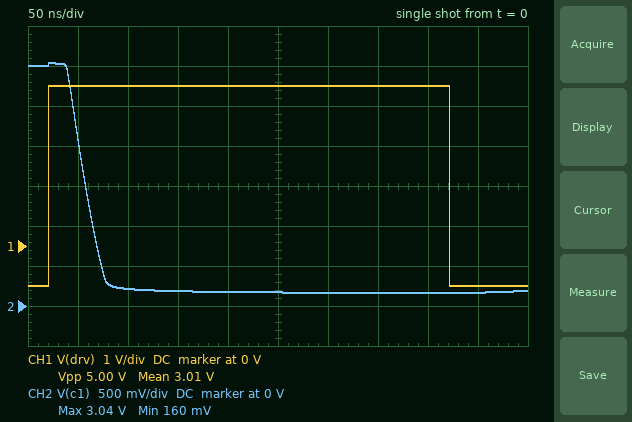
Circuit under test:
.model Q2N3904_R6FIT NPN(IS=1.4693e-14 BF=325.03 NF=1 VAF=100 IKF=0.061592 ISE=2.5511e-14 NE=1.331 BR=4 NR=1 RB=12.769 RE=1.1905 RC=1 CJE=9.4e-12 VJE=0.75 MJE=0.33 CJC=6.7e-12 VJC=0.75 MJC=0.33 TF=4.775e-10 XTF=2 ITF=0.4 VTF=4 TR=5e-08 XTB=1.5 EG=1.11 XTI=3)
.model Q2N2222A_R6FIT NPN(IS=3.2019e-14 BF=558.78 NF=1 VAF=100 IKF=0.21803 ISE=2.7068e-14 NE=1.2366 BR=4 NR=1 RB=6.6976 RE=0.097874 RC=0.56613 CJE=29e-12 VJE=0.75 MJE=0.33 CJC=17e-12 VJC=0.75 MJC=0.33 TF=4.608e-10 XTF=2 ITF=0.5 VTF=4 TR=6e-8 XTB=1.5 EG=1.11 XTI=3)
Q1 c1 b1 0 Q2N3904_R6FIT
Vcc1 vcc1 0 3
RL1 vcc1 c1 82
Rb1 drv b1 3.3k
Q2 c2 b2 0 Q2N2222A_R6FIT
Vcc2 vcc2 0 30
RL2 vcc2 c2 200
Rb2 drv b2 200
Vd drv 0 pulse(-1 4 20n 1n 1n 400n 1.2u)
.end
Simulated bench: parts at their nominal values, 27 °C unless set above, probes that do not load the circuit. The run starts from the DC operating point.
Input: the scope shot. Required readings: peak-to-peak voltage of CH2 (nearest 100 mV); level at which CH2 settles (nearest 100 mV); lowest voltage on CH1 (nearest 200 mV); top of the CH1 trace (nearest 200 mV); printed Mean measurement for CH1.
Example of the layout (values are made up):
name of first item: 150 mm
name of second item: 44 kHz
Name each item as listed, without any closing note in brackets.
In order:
peak-to-peak voltage of CH2: 2.9 V
level at which CH2 settles: 200 mV
lowest voltage on CH1: -1.0 V
top of the CH1 trace: 4.0 V
printed Mean measurement for CH1: 3.01 V
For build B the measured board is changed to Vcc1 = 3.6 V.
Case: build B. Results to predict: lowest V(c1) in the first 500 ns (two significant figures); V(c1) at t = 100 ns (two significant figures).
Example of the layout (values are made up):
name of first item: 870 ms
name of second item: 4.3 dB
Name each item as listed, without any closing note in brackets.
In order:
lowest V(c1) in the first 500 ns: 180 mV
V(c1) at t = 100 ns: 250 mV
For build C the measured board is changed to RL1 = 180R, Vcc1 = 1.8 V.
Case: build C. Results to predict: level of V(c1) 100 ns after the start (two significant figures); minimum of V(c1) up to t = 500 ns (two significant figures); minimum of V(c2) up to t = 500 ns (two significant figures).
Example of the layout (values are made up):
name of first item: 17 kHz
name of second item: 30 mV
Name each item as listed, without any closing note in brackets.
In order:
level of V(c1) 100 ns after the start: 97 mV
minimum of V(c1) up to t = 500 ns: 60 mV
minimum of V(c2) up to t = 500 ns: 150 mV
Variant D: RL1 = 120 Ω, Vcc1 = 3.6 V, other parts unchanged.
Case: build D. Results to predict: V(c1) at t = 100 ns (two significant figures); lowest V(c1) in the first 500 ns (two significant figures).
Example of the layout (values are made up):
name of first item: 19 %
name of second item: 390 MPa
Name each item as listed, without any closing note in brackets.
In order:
V(c1) at t = 100 ns: 190 mV
lowest V(c1) in the first 500 ns: 140 mV
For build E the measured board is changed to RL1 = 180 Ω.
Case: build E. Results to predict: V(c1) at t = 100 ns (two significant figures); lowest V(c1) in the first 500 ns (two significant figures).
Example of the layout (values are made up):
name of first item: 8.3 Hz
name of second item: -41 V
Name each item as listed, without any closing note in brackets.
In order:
V(c1) at t = 100 ns: 130 mV
lowest V(c1) in the first 500 ns: 89 mV
